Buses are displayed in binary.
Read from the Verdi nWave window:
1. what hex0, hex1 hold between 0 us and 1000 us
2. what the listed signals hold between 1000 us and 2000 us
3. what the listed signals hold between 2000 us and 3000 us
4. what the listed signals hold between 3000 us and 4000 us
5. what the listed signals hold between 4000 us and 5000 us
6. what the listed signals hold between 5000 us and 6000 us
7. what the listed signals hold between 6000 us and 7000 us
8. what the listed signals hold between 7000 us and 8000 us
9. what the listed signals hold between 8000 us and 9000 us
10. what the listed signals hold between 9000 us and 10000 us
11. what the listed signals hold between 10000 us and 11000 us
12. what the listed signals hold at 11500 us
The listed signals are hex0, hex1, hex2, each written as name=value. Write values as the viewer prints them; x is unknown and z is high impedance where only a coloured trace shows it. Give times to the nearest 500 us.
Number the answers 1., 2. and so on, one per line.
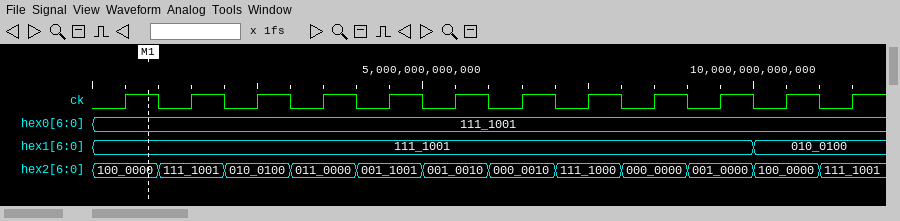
1. hex0=111_1001, hex1=111_1001
2. hex0=111_1001, hex1=111_1001, hex2=111_1001
3. hex0=111_1001, hex1=111_1001, hex2=010_0100
4. hex0=111_1001, hex1=111_1001, hex2=011_0000
5. hex0=111_1001, hex1=111_1001, hex2=001_1001
6. hex0=111_1001, hex1=111_1001, hex2=001_0010
7. hex0=111_1001, hex1=111_1001, hex2=000_0010
8. hex0=111_1001, hex1=111_1001, hex2=111_1000
9. hex0=111_1001, hex1=111_1001, hex2=000_0000
10. hex0=111_1001, hex1=111_1001, hex2=001_0000
11. hex0=111_1001, hex1=010_0100, hex2=100_0000
12. hex0=111_1001, hex1=010_0100, hex2=111_1001
